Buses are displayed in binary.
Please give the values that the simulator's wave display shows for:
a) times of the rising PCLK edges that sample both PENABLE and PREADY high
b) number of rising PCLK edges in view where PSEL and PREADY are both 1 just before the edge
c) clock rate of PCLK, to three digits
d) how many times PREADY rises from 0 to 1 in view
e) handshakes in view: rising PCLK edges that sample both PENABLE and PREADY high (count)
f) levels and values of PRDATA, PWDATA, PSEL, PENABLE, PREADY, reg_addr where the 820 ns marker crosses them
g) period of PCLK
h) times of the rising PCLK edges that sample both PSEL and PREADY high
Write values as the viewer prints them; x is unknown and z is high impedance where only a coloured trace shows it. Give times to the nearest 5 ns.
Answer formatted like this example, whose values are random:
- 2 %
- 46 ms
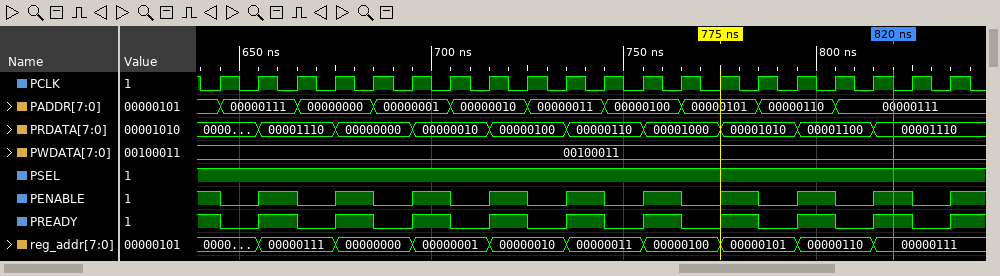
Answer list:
- 645 ns, 665 ns, 685 ns, 705 ns, 725 ns, 745 ns, 765 ns, 785 ns, 805 ns, 825 ns
- 10
- 100 MHz
- 10
- 10
- PRDATA=00001110, PWDATA=00100011, PSEL=1, PENABLE=1, PREADY=1, reg_addr=00000111
- 10 ns
- 645 ns, 665 ns, 685 ns, 705 ns, 725 ns, 745 ns, 765 ns, 785 ns, 805 ns, 825 ns
